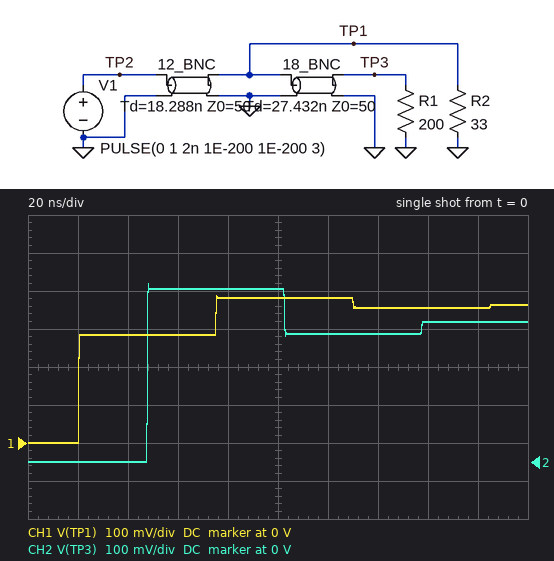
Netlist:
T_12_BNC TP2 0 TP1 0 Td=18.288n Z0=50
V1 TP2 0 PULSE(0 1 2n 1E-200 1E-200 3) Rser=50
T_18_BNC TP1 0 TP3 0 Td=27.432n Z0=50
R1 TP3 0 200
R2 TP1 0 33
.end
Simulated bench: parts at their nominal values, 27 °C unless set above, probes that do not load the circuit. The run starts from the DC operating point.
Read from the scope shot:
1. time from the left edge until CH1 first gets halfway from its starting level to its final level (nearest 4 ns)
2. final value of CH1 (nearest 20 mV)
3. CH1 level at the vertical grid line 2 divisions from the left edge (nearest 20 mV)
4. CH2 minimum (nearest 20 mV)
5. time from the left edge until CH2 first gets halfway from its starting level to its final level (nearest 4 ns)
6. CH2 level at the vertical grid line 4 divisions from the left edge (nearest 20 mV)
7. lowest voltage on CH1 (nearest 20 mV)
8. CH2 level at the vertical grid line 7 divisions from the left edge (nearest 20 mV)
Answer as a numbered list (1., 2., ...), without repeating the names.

1. 20 ns
2. 360 mV
3. 280 mV
4. 0 V
5. 48 ns
6. 460 mV
7. 0 V
8. 340 mV
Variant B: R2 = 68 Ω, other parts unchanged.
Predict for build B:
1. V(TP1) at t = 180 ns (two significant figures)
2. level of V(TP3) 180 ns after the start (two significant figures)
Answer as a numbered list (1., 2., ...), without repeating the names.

1. 500 mV
2. 510 mV
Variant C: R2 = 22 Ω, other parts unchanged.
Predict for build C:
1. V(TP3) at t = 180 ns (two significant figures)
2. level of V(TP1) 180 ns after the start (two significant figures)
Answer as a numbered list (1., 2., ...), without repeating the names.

1. 290 mV
2. 280 mV
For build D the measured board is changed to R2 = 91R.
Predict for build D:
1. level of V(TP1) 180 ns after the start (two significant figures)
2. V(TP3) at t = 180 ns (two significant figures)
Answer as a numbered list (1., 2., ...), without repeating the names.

1. 550 mV
2. 560 mV
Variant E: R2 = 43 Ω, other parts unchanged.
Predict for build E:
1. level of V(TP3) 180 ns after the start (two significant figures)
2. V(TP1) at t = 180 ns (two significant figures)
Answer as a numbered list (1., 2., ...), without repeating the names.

1. 420 mV
2. 410 mV
